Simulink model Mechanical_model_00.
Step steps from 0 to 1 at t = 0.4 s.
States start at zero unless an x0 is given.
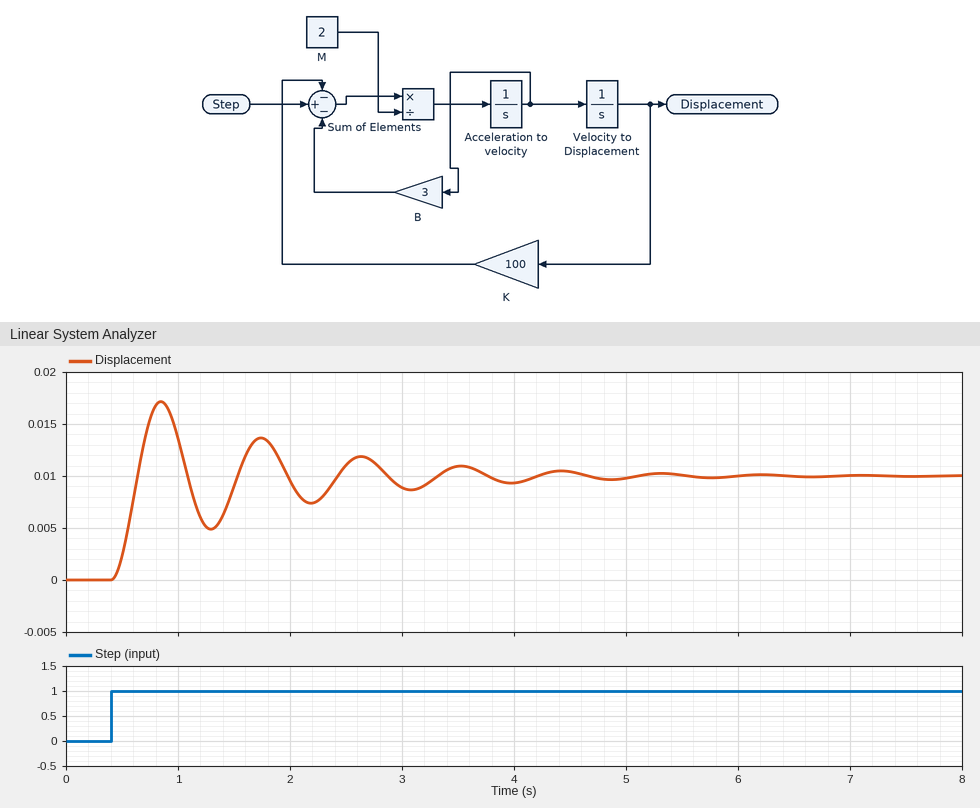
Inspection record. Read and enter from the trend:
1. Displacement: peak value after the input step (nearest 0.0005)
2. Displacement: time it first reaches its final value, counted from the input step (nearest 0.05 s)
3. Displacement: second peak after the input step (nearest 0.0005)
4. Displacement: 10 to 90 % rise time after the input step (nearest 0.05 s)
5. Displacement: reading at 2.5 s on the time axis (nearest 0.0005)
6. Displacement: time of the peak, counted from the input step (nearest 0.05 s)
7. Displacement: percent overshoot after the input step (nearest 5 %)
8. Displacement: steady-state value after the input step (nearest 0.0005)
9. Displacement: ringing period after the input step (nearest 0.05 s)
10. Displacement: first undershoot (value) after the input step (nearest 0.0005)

0.0170
0.25 s
0.0135
0.15 s
0.0110
0.45 s
70 %
0.0100
0.90 s
0.0050
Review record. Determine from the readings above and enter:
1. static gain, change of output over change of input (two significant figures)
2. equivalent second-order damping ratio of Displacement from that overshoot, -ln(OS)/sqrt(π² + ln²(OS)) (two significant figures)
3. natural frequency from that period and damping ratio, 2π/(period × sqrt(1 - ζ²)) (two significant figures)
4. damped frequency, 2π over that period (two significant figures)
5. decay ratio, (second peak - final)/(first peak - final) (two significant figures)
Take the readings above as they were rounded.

0.010
0.11
7.0 rad/s
7.0 rad/s
0.50
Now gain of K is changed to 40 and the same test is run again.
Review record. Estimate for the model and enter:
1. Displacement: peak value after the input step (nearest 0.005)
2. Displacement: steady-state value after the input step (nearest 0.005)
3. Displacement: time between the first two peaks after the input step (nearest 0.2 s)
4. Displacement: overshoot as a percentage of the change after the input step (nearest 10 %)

0.040
0.025
1.4 s
60 %
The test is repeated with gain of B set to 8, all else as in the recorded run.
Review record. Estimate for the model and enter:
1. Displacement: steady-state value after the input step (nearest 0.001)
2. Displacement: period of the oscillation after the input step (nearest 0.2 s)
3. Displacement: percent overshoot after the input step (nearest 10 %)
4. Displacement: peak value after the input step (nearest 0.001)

0.010
1.0 s
40 %
0.014
